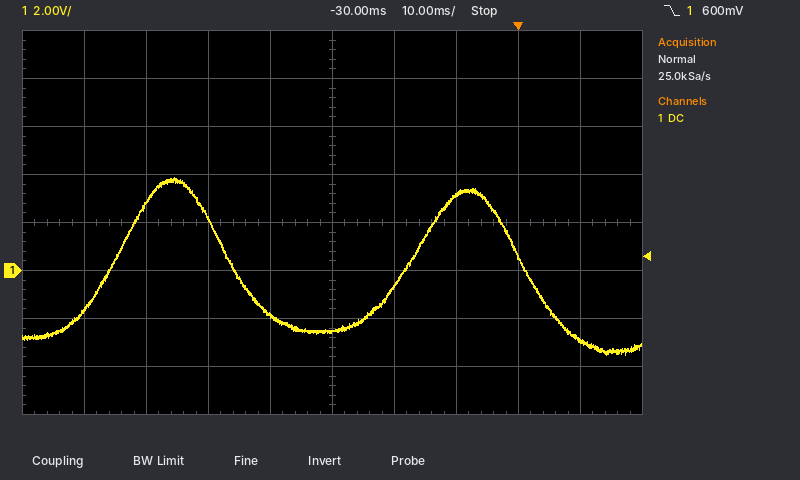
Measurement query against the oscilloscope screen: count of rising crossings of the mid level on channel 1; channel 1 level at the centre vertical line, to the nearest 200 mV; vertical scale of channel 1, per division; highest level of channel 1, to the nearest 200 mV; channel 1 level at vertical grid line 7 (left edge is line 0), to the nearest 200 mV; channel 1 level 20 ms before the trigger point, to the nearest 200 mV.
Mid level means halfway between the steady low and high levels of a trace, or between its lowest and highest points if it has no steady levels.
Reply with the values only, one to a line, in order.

2
-2.6 V
2 V
3.8 V
3.2 V
-600 mV
